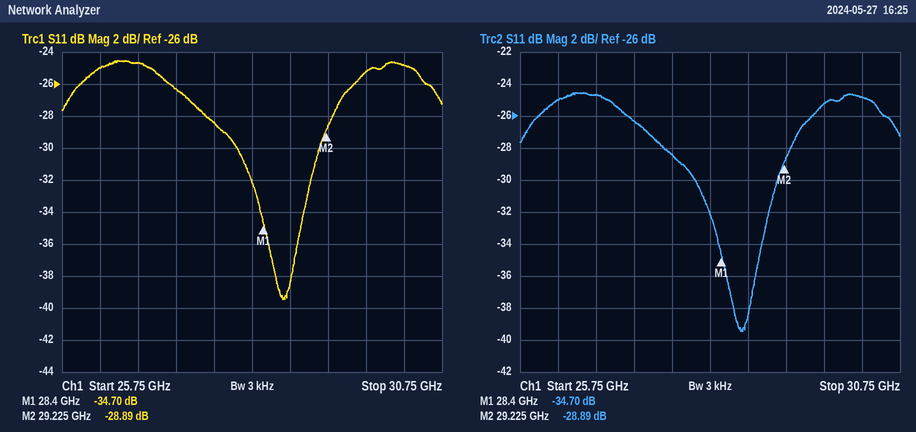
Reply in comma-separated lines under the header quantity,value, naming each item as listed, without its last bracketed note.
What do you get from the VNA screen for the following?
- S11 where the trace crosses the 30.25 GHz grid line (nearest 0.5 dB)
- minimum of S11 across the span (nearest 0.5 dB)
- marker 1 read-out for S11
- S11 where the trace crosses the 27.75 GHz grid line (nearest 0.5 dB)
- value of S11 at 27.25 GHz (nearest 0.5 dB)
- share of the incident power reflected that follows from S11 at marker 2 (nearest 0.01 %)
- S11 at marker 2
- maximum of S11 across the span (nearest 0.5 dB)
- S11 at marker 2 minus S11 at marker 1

quantity,value
S11 where the trace crosses the 30.25 GHz grid line,-25.0 dB
minimum of S11 across the span,-39.5 dB
marker 1 read-out for S11,-34.70 dB
S11 where the trace crosses the 27.75 GHz grid line,-28.5 dB
value of S11 at 27.25 GHz,-26.5 dB
share of the incident power reflected that follows from S11 at marker 2,0.13 %
S11 at marker 2,-28.89 dB
maximum of S11 across the span,-24.5 dB
S11 at marker 2 minus S11 at marker 1,5.81 dB
